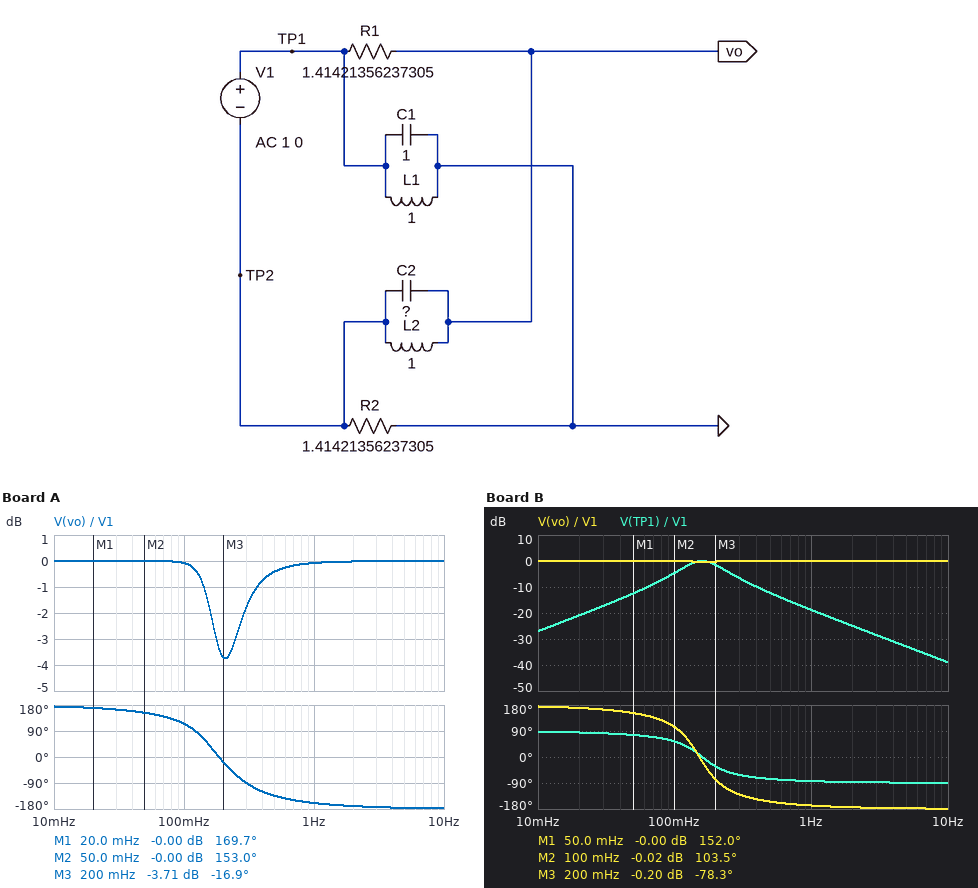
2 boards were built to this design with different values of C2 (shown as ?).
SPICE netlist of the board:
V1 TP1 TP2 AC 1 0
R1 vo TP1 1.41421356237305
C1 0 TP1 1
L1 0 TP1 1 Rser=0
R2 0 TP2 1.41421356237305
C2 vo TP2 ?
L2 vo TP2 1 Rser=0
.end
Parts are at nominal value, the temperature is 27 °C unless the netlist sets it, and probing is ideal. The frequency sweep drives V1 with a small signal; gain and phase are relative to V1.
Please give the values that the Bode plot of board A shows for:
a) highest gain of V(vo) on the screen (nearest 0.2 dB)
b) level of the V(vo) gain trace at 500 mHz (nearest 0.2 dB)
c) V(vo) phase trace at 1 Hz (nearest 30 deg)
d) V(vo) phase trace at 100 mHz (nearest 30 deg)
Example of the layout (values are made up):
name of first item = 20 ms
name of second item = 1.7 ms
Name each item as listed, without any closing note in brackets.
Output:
highest gain of V(vo) on the screen = 0 dB
level of the V(vo) gain trace at 500 mHz = -0.4 dB
V(vo) phase trace at 1 Hz = -150 deg
V(vo) phase trace at 100 mHz = 120 deg
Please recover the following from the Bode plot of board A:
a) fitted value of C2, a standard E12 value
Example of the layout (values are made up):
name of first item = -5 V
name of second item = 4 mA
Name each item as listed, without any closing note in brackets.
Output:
fitted value of C2, a standard E12 value = 470 mF
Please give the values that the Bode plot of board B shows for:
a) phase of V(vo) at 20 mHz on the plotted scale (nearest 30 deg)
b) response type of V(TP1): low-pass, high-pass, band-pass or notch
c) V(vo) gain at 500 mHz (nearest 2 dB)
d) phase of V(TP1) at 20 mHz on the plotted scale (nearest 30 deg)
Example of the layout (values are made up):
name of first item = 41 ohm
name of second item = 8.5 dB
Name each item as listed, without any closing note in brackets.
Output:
phase of V(vo) at 20 mHz on the plotted scale = 180 deg
response type of V(TP1): low-pass, high-pass, band-pass or notch = band-pass
V(vo) gain at 500 mHz = 0 dB
phase of V(TP1) at 20 mHz on the plotted scale = 90 deg
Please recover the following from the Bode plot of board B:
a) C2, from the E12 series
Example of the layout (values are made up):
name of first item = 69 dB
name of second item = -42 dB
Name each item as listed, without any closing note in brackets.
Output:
C2, from the E12 series = 1.2 F
